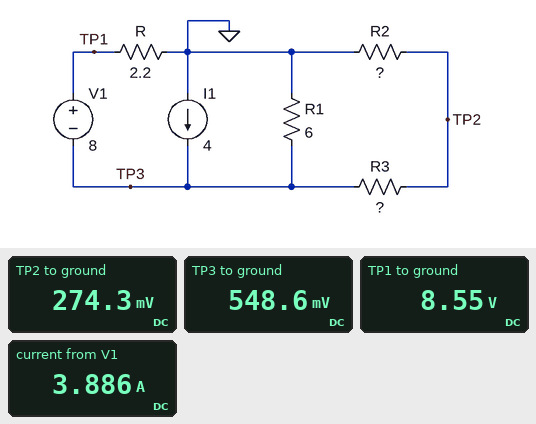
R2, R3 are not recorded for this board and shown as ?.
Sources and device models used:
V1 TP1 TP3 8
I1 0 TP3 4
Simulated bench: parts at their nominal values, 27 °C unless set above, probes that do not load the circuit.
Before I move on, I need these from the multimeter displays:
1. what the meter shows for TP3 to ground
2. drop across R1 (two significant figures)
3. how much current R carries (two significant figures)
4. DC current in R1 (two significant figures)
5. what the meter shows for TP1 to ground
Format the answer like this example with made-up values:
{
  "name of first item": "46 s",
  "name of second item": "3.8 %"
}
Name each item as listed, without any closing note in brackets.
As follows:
{
  "what the meter shows for TP3 to ground": "548.6 mV",
  "drop across R1": "550 mV",
  "how much current R carries": "3.9 A",
  "DC current in R1": "91 mA",
  "what the meter shows for TP1 to ground": "8.55 V"
}
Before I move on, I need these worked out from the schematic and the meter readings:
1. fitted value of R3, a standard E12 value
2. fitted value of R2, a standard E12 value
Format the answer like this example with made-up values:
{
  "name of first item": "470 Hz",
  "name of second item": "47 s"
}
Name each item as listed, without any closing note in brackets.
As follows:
{
  "fitted value of R3, a standard E12 value": "12 Ω",
  "fitted value of R2, a standard E12 value": "12 Ω"
}
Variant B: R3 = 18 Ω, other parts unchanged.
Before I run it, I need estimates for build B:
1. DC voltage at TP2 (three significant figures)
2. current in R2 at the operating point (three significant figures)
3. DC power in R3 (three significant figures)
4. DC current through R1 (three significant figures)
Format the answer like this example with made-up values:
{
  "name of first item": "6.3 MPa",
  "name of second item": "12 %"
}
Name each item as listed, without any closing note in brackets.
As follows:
{
  "DC voltage at TP2": "222 mV",
  "current in R2 at the operating point": "18.5 mA",
  "DC power in R3": "6.17 mW",
  "DC current through R1": "92.6 mA"
}
